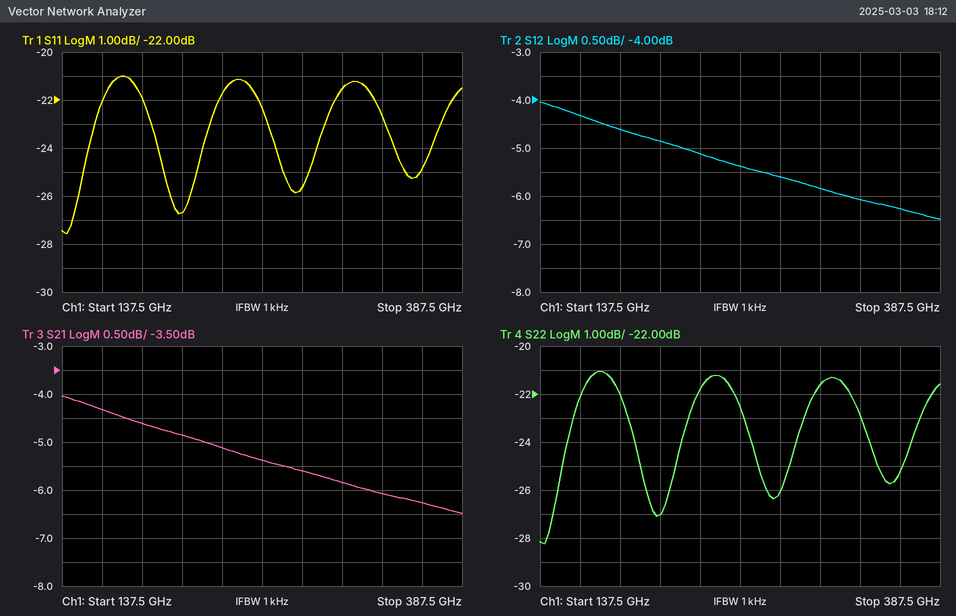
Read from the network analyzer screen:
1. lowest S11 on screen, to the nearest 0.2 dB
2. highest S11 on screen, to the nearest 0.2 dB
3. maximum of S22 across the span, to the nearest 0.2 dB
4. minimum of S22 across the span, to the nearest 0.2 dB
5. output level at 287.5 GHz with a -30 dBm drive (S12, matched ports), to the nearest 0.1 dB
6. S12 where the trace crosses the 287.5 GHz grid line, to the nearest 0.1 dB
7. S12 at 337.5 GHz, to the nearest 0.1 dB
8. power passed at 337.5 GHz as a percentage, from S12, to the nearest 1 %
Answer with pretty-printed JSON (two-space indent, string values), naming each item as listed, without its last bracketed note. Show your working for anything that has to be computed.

{
  "lowest S11 on screen, to the nearest 0.2 dB": "-27.6 dB",
  "highest S11 on screen, to the nearest 0.2 dB": "-21.0 dB",
  "maximum of S22 across the span, to the nearest 0.2 dB": "-21.0 dB",
  "minimum of S22 across the span, to the nearest 0.2 dB": "-28.2 dB",
  "output level at 287.5 GHz with a -30 dBm drive (S12, matched ports), to the nearest 0.1 dB": "-30 dBm + (-5.6 dB) = -35.6 dBm",
  "S12 where the trace crosses the 287.5 GHz grid line, to the nearest 0.1 dB": "-5.6 dB",
  "S12 at 337.5 GHz, to the nearest 0.1 dB": "-6.1 dB",
  "power passed at 337.5 GHz as a percentage, from S12, to the nearest 1 %": "10^(-6.1/10) ≈ 25 %"
}
